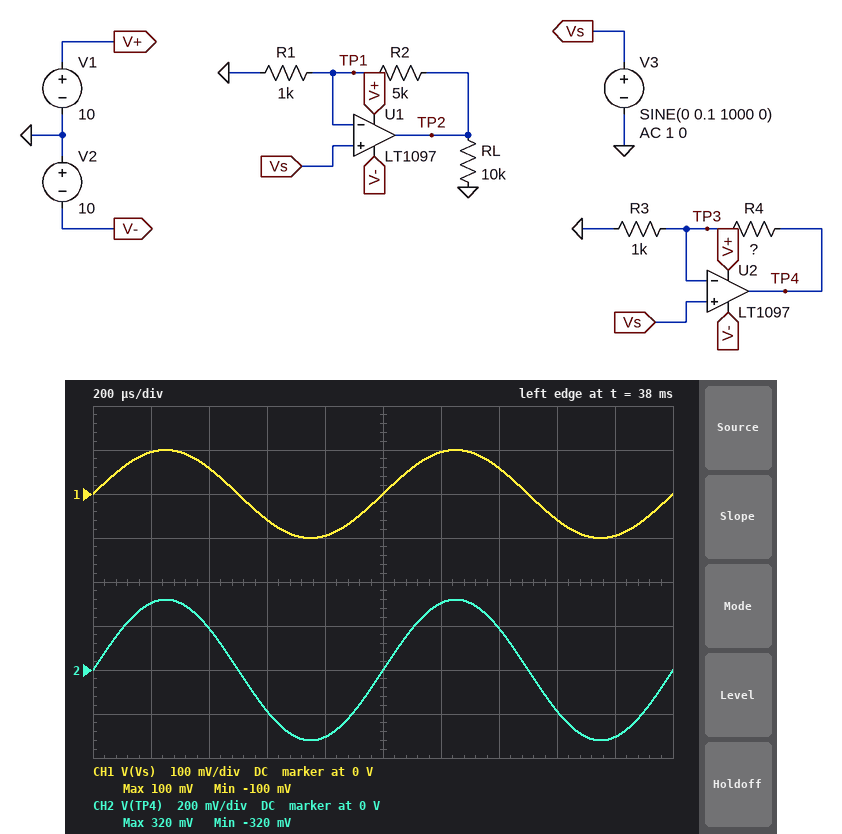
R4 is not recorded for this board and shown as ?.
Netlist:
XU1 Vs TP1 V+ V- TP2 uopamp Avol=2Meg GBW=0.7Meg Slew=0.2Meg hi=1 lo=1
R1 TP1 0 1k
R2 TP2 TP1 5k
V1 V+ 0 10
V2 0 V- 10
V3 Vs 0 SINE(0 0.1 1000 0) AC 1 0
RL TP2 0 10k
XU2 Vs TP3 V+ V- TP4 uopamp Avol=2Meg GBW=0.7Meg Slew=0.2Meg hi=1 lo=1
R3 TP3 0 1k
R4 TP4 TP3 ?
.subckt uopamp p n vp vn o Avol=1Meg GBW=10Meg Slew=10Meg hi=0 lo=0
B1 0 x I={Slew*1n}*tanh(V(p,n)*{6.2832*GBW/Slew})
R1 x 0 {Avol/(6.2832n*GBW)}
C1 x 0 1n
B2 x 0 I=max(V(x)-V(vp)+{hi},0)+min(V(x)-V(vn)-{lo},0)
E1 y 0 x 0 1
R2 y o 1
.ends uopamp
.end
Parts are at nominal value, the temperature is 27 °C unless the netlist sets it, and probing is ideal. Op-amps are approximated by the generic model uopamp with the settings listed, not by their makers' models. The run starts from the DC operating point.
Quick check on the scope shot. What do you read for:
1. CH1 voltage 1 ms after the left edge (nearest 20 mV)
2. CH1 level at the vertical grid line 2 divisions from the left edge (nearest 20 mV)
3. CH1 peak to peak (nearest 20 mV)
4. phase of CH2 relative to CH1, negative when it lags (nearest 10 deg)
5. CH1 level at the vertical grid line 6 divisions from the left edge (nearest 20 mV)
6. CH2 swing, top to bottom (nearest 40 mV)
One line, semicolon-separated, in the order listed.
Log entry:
0 V; 60 mV; 200 mV; 0 deg; 100 mV; 640 mV
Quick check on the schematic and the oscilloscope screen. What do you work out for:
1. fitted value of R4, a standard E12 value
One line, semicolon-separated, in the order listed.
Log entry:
2.2 kΩ
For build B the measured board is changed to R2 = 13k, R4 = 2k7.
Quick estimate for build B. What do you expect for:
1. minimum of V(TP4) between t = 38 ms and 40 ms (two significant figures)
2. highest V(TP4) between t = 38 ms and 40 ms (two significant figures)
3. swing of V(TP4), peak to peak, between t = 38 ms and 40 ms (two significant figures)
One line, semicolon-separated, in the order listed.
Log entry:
-370 mV; 370 mV; 740 mV
